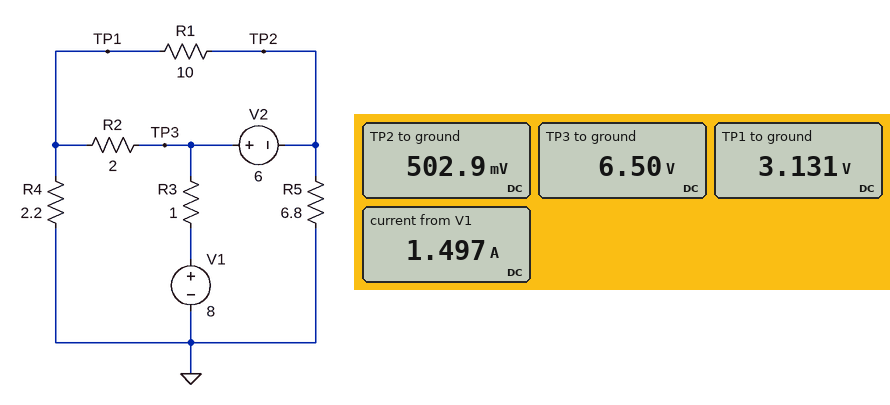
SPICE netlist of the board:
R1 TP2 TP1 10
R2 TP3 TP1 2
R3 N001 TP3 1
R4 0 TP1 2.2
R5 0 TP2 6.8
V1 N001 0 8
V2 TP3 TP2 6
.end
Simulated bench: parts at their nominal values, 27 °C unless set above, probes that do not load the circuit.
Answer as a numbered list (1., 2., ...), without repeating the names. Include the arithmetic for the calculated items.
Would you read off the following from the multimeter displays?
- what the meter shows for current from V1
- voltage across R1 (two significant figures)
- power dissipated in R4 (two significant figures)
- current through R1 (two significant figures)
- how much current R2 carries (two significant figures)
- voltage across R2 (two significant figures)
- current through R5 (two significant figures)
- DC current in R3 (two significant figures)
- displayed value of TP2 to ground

1. 1.497 A
2. 3.131 V - 502.9 mV = 2.6 V
3. (3.131 V)^2 / 2.2 Ω = 4.5 W
4. (3.131 V - 502.9 mV) / 10 Ω = 260 mA
5. (6.5 V - 3.131 V) / 2 Ω = 1.7 A
6. 6.5 V - 3.131 V = 3.4 V
7. (502.9 mV) / 6.8 Ω = 74 mA
8. (8 V - 6.5 V) / 1 Ω = 1.5 A
9. 502.9 mV
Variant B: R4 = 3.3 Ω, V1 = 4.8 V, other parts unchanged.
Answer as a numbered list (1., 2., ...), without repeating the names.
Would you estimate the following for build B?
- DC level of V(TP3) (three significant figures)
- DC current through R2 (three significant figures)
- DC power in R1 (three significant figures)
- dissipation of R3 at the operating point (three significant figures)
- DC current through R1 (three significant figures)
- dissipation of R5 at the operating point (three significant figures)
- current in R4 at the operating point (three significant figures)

1. 4.36 V
2. 1.06 A
3. 1.50 W
4. 191 mW
5. 387 mA
6. 394 mW
7. 677 mA
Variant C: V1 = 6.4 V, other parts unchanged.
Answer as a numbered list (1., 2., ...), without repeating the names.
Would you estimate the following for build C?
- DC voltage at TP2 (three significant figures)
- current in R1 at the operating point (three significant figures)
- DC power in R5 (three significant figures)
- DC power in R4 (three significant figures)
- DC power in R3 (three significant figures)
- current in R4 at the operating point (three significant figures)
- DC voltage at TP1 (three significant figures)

1. -635 mV
2. 312 mA
3. 59.4 mW
4. 2.80 W
5. 1.07 W
6. 1.13 A
7. 2.48 V
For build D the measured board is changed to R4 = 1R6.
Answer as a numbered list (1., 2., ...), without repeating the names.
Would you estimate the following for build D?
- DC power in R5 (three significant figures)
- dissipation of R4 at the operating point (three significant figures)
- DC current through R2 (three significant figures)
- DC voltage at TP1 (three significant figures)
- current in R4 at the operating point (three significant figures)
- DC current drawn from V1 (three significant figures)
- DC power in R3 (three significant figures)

1. 15.3 mW
2. 4.25 W
3. 1.86 A
4. 2.61 V
5. 1.63 A
6. 1.68 A
7. 2.81 W
